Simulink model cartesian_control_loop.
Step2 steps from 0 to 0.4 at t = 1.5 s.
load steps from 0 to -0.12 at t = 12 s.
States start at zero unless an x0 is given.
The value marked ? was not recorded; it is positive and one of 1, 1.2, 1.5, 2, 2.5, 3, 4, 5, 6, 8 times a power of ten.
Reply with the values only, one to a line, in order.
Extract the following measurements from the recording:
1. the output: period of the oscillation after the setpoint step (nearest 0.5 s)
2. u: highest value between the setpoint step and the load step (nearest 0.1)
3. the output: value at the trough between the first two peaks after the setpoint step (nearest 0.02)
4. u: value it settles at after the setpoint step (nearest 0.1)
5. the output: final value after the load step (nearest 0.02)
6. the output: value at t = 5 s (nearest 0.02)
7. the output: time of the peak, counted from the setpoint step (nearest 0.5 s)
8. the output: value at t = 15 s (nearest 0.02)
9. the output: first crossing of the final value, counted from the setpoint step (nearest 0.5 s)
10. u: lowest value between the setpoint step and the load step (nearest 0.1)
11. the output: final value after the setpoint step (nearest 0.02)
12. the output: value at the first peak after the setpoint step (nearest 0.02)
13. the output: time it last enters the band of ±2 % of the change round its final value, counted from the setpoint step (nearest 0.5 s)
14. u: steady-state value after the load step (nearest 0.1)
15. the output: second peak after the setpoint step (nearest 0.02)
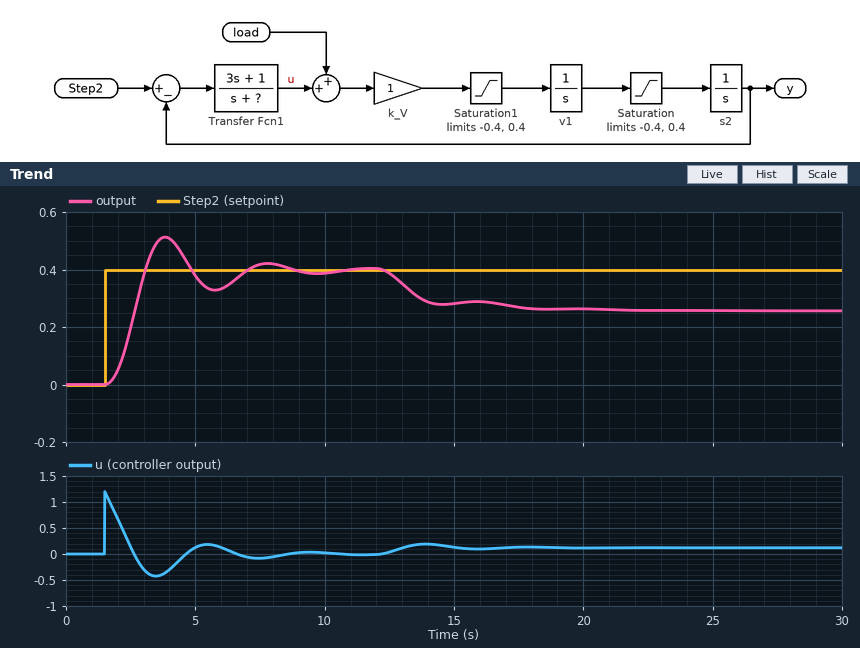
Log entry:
4.0 s
1.2
0.32
0.0
0.26
0.38
2.5 s
0.28
1.5 s
-0.4
0.40
0.52
9.0 s
0.1
0.42
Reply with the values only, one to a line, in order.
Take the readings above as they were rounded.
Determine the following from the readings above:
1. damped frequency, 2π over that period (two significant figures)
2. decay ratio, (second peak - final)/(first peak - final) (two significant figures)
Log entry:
1.6 rad/s
0.17
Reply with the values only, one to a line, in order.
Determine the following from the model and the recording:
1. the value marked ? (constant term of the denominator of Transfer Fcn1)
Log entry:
1.2
